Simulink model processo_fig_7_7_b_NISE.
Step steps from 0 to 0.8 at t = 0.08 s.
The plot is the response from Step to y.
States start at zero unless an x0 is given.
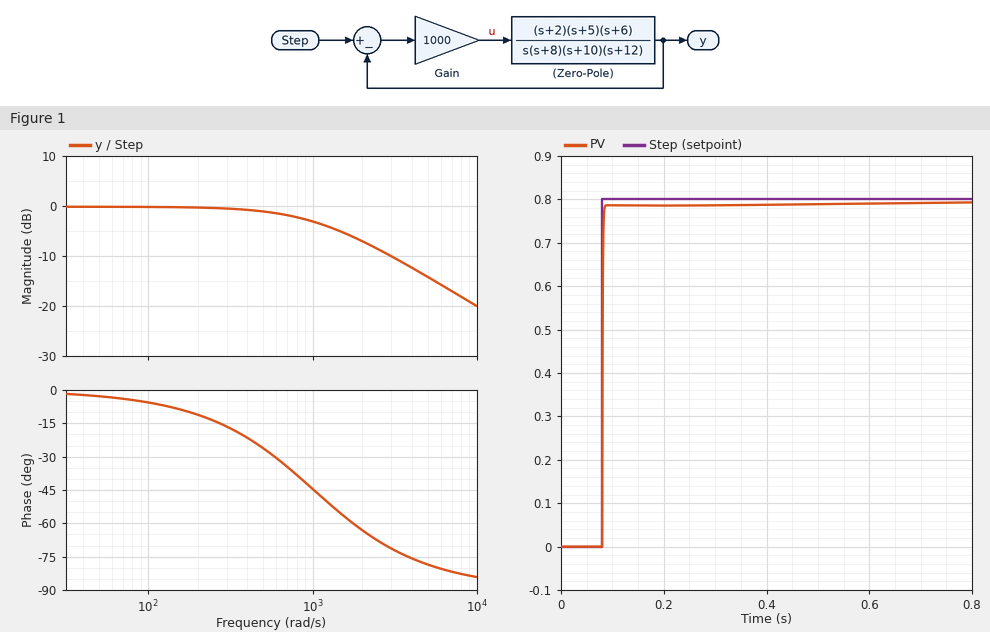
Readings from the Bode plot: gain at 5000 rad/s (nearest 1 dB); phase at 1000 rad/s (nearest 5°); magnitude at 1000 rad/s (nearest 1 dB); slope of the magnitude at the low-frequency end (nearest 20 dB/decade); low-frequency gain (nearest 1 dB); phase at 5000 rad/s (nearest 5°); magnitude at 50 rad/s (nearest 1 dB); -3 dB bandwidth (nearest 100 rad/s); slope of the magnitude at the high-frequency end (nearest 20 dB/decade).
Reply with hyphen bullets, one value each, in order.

- -14 dB
- -45°
- -3 dB
- 0 dB/decade
- 0 dB
- -80°
- 0 dB
- 1000 rad/s
- -20 dB/decade
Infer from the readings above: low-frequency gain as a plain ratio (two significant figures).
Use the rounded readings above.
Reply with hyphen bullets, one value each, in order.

- 1.0
